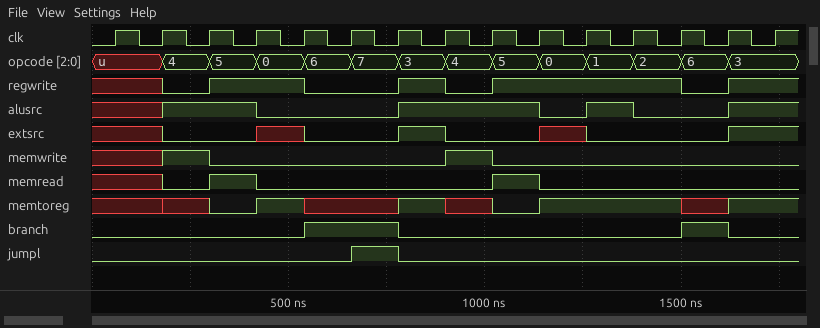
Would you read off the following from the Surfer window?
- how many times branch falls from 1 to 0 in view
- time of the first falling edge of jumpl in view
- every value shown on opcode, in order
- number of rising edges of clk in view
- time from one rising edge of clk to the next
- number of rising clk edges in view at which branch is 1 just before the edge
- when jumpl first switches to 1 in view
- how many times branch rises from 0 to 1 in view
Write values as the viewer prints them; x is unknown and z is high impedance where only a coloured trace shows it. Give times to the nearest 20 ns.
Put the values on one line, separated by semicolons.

2; 780 ns; u, 4, 5, 0, 6, 7, 3, 4, 5, 0, 1, 2, 6, 3; 15; 120 ns; 3; 660 ns; 2
